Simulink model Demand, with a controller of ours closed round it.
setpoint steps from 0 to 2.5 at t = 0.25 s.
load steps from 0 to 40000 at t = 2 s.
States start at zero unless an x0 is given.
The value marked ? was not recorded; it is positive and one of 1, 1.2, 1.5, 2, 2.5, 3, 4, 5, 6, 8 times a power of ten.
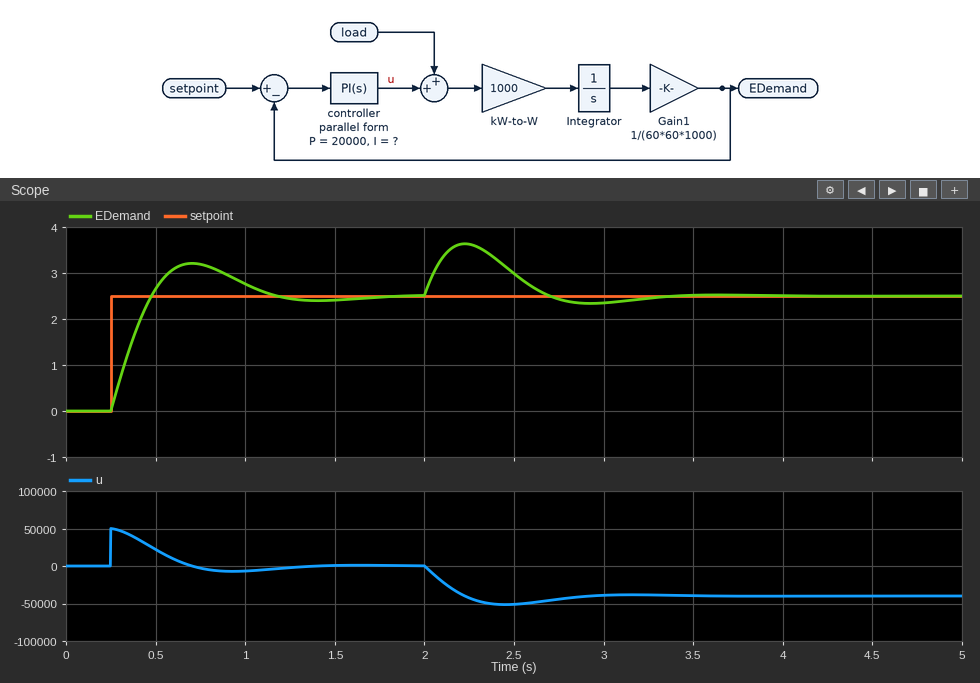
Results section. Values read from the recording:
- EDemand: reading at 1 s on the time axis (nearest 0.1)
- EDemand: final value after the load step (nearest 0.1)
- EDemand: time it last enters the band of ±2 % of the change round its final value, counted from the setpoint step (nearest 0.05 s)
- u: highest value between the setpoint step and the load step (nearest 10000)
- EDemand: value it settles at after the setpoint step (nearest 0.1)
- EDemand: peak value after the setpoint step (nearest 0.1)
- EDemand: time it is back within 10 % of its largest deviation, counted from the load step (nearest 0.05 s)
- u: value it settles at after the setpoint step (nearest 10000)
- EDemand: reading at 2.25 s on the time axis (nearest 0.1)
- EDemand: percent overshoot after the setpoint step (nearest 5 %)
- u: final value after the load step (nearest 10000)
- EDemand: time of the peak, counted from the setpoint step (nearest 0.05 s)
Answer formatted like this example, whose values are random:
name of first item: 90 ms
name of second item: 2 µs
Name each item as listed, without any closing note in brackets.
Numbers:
EDemand: reading at 1 s on the time axis: 2.8
EDemand: final value after the load step: 2.5
EDemand: time it last enters the band of ±2 % of the change round its final value, counted from the setpoint step: 1.40 s
u: highest value between the setpoint step and the load step: 50000
EDemand: value it settles at after the setpoint step: 2.5
EDemand: peak value after the setpoint step: 3.2
EDemand: time it is back within 10 % of its largest deviation, counted from the load step: 1.10 s
u: value it settles at after the setpoint step: 0
EDemand: reading at 2.25 s on the time axis: 3.6
EDemand: percent overshoot after the setpoint step: 30 %
u: final value after the load step: -40000
EDemand: time of the peak, counted from the setpoint step: 0.45 s
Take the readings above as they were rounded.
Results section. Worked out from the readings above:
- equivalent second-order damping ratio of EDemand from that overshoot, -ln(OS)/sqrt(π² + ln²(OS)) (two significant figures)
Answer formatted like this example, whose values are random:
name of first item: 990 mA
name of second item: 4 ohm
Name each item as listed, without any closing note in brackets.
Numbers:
equivalent second-order damping ratio of EDemand from that overshoot, -ln(OS)/sqrt(π² + ln²(OS)): 0.36
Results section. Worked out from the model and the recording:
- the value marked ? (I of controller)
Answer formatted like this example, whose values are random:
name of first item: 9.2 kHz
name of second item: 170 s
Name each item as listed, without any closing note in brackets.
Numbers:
the value marked ?: 100000
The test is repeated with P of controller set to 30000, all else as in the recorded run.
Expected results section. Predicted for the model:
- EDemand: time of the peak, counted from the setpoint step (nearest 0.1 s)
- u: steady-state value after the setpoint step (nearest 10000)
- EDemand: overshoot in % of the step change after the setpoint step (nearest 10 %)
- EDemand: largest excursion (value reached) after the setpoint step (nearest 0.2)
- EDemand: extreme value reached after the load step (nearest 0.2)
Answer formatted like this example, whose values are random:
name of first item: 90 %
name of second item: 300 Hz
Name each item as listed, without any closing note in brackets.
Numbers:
EDemand: time of the peak, counted from the setpoint step: 0.4 s
u: steady-state value after the setpoint step: 0
EDemand: overshoot in % of the step change after the setpoint step: 20 %
EDemand: largest excursion (value reached) after the setpoint step: 3.0
EDemand: extreme value reached after the load step: 3.4
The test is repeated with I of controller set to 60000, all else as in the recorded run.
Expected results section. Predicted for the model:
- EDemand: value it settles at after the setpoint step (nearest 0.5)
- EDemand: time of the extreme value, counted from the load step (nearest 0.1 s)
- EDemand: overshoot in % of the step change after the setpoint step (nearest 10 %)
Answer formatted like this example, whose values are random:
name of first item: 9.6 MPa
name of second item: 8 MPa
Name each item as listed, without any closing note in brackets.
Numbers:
EDemand: value it settles at after the setpoint step: 2.5
EDemand: time of the extreme value, counted from the load step: 0.3 s
EDemand: overshoot in % of the step change after the setpoint step: 20 %
